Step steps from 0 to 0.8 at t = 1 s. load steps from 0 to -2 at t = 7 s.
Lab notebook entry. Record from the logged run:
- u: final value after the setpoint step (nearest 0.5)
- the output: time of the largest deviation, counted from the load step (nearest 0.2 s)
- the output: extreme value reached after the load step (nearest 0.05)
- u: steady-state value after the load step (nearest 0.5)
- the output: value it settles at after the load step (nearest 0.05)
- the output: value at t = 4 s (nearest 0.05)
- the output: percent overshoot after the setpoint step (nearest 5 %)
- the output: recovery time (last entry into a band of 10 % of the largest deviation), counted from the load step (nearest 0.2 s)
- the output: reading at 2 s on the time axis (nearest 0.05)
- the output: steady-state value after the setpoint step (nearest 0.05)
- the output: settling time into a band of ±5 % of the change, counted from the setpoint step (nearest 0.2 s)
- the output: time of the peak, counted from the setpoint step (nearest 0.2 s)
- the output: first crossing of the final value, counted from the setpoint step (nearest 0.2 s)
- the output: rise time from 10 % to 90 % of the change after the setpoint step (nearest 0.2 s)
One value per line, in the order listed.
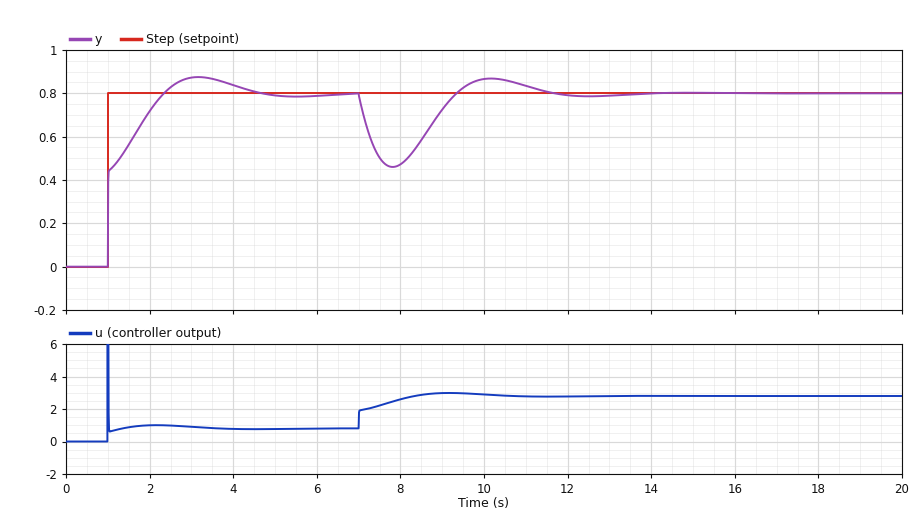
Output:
1.0
0.8 s
0.45
3.0
0.80
0.85
10 %
4.0 s
0.70
0.80
3.0 s
2.2 s
1.4 s
1.0 s
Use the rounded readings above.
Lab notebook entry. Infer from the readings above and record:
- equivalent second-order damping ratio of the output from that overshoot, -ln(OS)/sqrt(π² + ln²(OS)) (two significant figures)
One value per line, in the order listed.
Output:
0.59
